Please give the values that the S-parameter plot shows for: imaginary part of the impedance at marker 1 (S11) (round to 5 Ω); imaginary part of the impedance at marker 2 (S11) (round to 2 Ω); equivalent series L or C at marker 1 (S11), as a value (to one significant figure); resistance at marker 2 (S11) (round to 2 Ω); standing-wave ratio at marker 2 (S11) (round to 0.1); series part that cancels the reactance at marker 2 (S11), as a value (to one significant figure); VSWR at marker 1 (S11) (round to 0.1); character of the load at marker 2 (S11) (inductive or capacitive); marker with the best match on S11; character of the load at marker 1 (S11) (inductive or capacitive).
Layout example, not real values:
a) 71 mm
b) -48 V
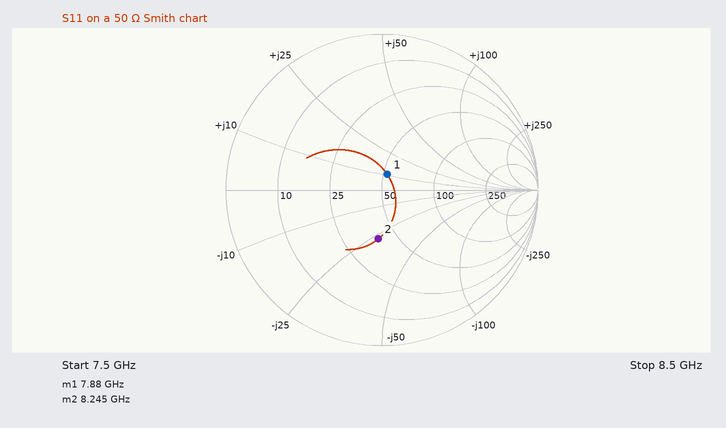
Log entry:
a) +10 Ω
b) -28 Ω
c) 200 pH
d) 40 Ω
e) 1.9
f) 500 pH
g) 1.2
h) capacitive
i) marker 1
j) inductive
